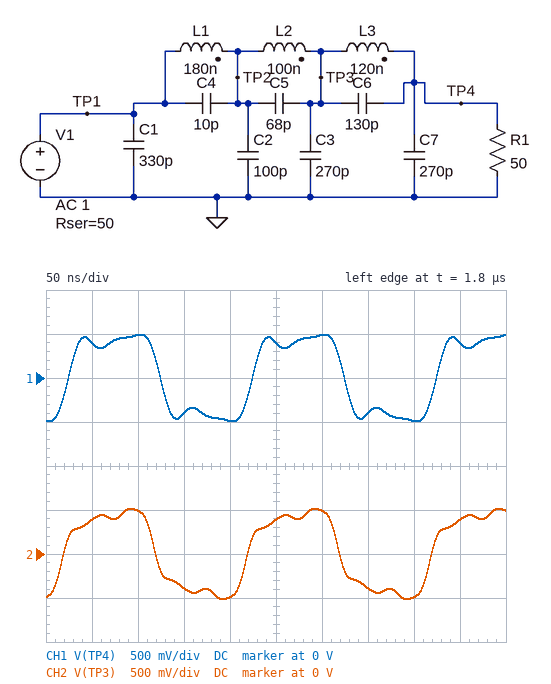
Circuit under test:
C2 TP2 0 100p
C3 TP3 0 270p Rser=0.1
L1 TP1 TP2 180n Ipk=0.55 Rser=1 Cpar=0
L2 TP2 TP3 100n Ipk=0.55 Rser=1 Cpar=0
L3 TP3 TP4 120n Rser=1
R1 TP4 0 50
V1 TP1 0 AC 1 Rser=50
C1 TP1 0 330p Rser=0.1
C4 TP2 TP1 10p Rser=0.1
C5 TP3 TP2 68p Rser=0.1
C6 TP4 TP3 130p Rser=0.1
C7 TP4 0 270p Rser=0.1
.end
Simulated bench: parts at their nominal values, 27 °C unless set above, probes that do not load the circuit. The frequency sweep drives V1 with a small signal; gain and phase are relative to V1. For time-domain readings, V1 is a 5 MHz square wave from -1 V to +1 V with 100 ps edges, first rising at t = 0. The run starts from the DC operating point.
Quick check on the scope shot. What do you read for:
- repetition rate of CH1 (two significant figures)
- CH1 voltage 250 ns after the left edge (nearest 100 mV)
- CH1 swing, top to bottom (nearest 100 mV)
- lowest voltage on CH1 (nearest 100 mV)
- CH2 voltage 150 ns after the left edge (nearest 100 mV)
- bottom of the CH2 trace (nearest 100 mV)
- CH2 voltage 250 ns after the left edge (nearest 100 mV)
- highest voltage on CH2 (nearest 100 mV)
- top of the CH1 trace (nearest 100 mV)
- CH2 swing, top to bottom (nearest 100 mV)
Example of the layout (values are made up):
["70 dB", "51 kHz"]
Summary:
["5.0 MHz", "400 mV", "1.0 V", "-500 mV", "-400 mV", "-500 mV", "400 mV", "500 mV", "500 mV", "1.0 V"]
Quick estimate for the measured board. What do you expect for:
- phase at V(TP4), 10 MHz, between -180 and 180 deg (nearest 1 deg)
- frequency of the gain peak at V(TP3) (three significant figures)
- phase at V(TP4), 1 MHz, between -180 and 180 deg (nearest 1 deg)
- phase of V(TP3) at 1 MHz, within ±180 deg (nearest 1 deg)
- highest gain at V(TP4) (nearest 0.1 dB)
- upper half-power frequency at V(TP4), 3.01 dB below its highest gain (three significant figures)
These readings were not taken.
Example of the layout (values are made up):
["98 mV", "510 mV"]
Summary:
["-79 deg", "29.6 MHz", "-10 deg", "-9 deg", "-6.3 dB", "21.4 MHz"]
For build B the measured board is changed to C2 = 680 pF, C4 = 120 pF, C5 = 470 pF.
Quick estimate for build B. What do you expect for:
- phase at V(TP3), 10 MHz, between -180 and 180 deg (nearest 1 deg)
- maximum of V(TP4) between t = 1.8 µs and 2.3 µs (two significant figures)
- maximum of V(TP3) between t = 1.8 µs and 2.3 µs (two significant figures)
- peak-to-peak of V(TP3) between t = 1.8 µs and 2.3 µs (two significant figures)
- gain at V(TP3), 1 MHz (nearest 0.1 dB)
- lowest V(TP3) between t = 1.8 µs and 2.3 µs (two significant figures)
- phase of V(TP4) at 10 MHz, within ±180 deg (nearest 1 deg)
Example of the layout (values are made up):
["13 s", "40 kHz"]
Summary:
["-86 deg", "460 mV", "450 mV", "900 mV", "-6.3 dB", "-450 mV", "-98 deg"]
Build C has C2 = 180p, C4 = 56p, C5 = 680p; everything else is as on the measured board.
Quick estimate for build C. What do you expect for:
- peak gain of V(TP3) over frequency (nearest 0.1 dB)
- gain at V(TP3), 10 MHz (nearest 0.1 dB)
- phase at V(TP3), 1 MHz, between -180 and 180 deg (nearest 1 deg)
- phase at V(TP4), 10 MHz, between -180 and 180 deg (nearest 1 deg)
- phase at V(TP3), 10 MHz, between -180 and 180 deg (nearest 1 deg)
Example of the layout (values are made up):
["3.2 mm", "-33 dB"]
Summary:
["-6.1 dB", "-9.7 dB", "-10 deg", "-85 deg", "-74 deg"]
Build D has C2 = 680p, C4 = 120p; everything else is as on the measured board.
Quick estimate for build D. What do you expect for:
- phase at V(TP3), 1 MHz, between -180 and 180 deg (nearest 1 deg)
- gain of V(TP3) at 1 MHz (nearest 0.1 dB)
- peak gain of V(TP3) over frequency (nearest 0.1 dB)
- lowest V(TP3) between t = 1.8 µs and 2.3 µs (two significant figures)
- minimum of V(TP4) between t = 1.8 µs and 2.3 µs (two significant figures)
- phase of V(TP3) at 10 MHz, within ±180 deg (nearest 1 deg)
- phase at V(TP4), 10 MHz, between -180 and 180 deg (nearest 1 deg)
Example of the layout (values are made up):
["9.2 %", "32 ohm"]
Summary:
["-15 deg", "-6.3 dB", "-6.1 dB", "-440 mV", "-470 mV", "-84 deg", "-96 deg"]
